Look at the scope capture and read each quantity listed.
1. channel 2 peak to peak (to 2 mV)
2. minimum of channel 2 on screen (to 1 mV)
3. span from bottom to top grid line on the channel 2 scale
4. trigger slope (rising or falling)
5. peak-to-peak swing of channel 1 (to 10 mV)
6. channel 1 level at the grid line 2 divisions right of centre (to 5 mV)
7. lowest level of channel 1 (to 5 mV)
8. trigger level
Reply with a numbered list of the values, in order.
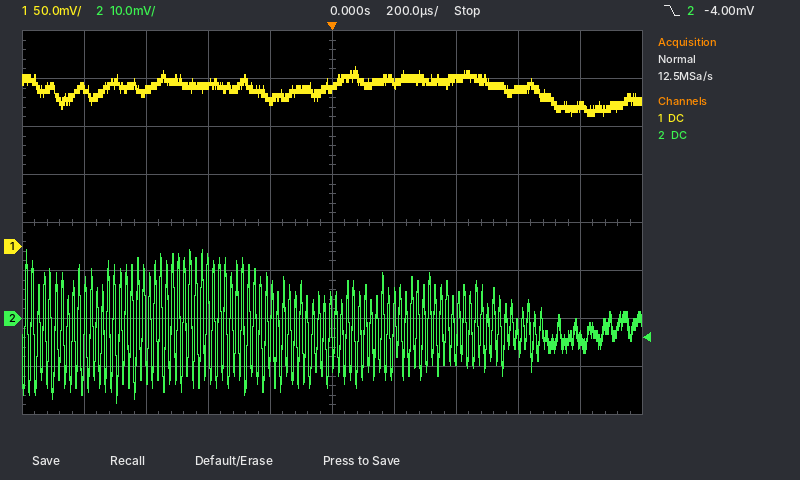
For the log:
1. 32 mV
2. -18 mV
3. 80 mV
4. falling
5. 50 mV
6. 175 mV
7. 135 mV
8. -4.00 mV
